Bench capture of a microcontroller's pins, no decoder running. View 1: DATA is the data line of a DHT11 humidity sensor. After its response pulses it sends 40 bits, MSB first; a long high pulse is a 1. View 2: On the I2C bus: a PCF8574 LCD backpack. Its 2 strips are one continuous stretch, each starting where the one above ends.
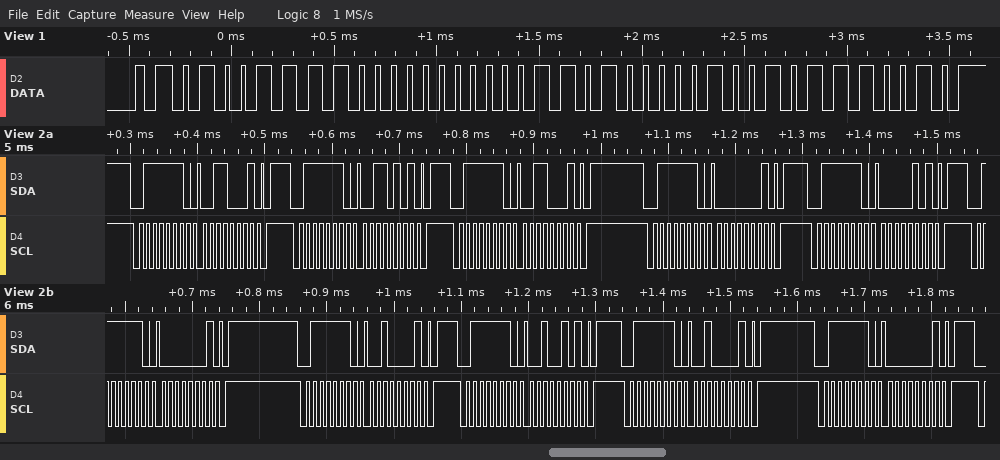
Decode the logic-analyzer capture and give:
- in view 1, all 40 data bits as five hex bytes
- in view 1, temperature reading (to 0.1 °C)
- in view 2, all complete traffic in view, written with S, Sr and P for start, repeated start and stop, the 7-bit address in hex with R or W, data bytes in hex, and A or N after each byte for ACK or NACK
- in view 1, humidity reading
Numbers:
4F 00 1A 09 72
26.9 °C
S 3FW A 31 A P S 3FW A 35 A P S 3FW A 31 A P S 3FW A 01 A P S 3FW A 05 A P S 3FW A 01 A P S 3FW A 21 A P S 3FW A 25 A P S 3FW A 21 A P S 3FW A 01 A P
79 %
